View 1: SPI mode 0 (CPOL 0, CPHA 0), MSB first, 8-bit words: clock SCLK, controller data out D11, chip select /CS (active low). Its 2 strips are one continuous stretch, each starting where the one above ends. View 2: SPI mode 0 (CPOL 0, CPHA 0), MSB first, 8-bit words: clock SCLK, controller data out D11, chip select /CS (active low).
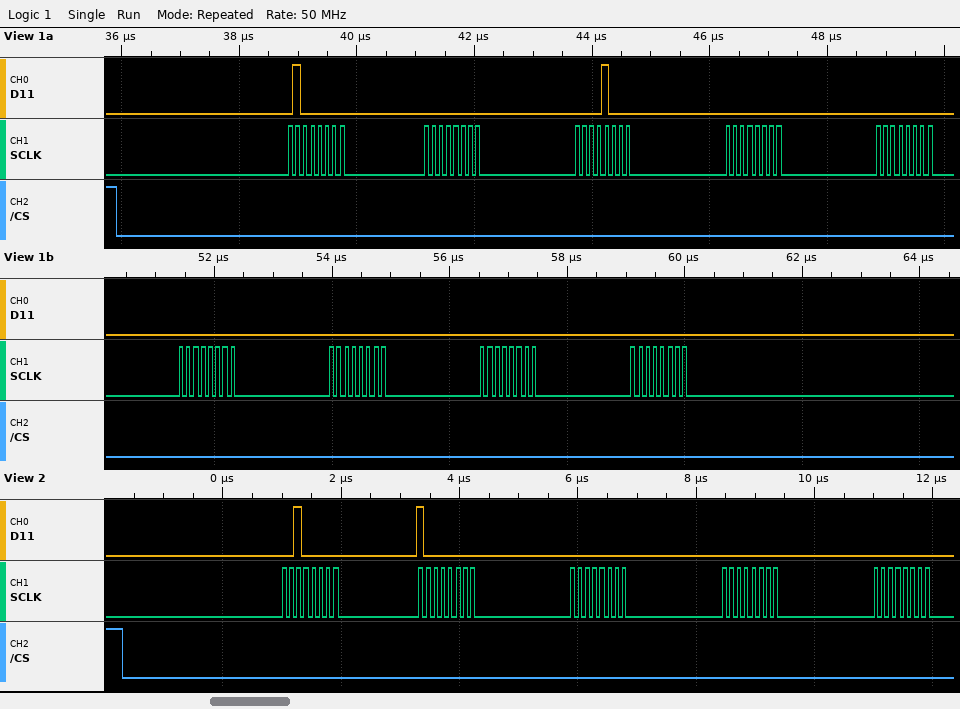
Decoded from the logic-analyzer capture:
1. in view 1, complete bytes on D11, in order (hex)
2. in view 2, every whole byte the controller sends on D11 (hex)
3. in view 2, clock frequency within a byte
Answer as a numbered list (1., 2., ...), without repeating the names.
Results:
1. 40 00 08 00 00 00 00 00 00
2. 20 80 00 00 00
3. 8 MHz
